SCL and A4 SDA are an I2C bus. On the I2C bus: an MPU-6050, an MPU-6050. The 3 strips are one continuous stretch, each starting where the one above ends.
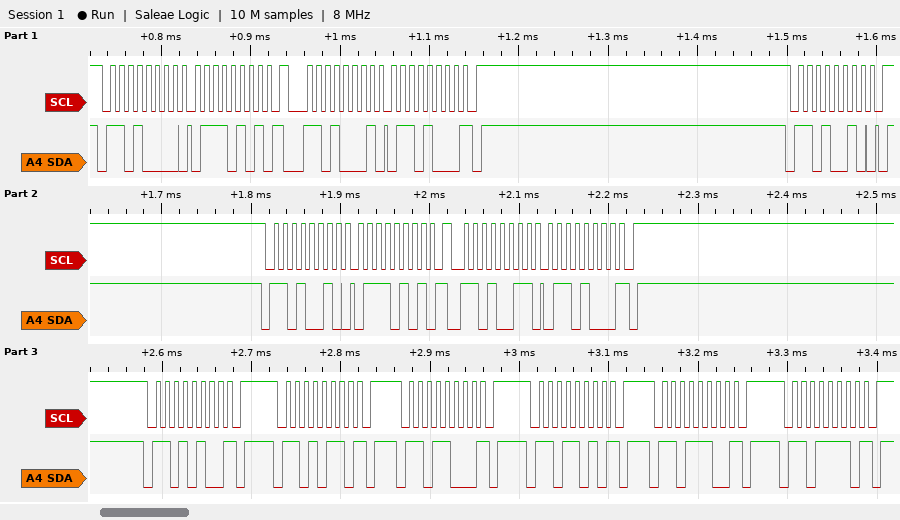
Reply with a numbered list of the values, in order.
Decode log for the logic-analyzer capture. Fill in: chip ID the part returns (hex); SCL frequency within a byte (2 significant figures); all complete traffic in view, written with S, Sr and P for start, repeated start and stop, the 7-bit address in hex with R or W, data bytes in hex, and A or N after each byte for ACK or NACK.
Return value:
1. 0x68
2. 100 kHz
3. S 68W A 75 A Sr 68R A 68 N P S 69W A P S 69W A 75 A Sr 69R A 68 N P S 6AW N P S 6BW N P S 6CW N P S 6DW N P S 6EW N P S 6FW N P
